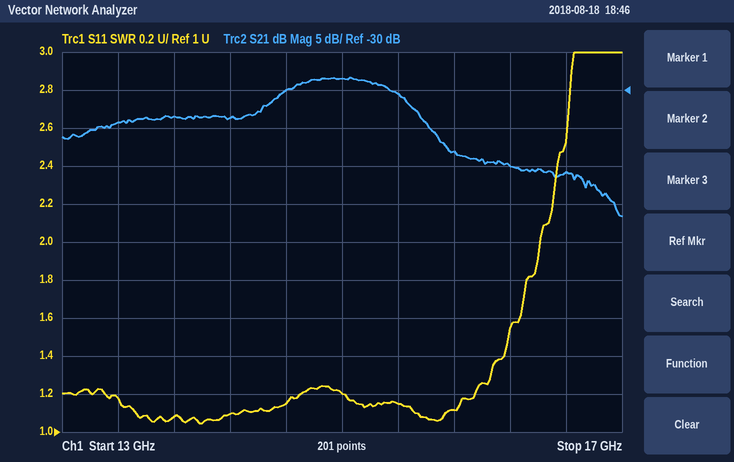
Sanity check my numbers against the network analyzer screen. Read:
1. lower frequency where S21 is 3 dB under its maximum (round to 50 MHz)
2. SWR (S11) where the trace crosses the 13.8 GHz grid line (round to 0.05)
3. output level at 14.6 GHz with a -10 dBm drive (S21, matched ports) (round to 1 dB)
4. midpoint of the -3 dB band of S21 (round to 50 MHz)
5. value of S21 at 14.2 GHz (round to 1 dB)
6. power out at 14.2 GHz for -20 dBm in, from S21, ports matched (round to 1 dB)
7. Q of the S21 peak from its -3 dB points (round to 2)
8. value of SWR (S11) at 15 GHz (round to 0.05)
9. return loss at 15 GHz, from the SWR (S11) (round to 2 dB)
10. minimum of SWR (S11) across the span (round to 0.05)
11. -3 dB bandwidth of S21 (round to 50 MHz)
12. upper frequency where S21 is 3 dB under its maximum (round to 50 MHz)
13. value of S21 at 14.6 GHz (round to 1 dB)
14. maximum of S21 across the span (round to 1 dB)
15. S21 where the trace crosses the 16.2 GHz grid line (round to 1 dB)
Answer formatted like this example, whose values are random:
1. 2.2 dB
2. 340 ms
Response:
1. 14.50 GHz
2. 1.10
3. -40 dBm
4. 15.00 GHz
5. -34 dB
6. -54 dBm
7. 16
8. 1.20
9. 20 dB
10. 1.05
11. 950 MHz
12. 15.45 GHz
13. -30 dB
14. -28 dB
15. -40 dB
